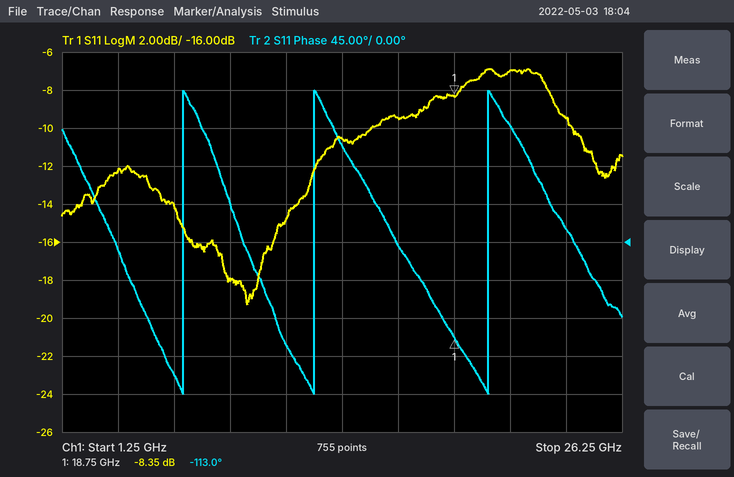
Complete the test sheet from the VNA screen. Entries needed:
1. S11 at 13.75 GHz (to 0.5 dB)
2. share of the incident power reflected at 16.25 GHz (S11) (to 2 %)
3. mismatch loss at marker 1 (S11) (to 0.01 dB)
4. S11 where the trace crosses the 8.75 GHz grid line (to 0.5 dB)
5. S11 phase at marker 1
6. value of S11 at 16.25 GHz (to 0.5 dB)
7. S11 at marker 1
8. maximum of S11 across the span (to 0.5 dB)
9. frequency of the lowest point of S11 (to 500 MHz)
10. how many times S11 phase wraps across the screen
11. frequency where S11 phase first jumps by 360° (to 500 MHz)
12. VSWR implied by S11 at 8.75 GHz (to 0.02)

-10.5 dB
12 %
0.69 dB
-18.0 dB
-113.0°
-9.5 dB
-8.35 dB
-7.0 dB
9.5 GHz
3
6.5 GHz
1.28
